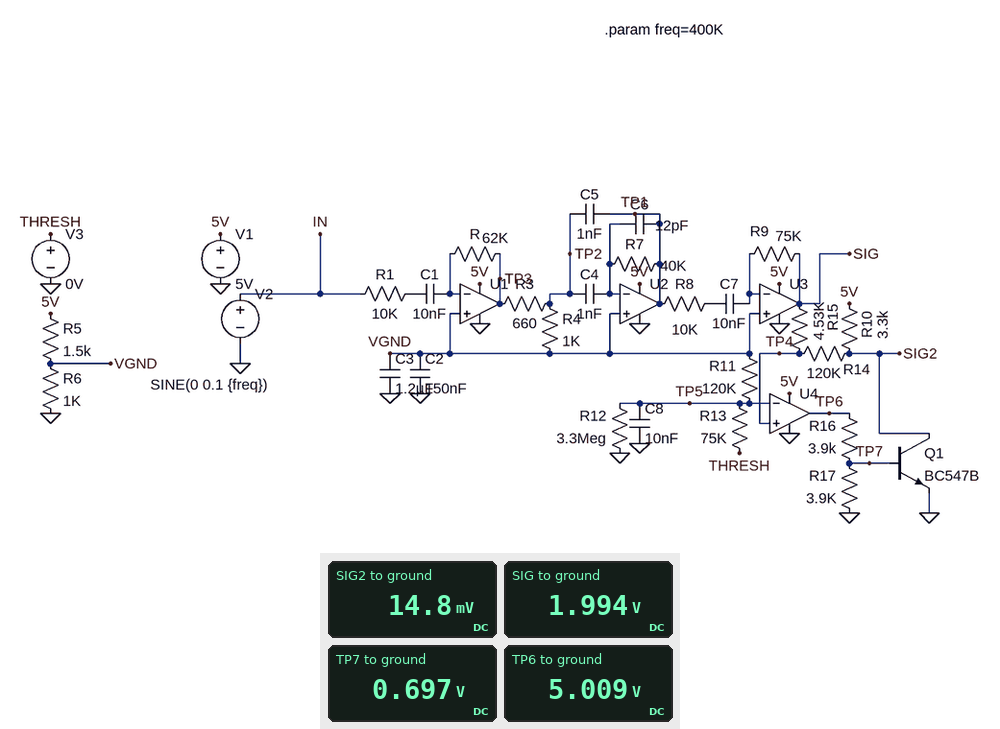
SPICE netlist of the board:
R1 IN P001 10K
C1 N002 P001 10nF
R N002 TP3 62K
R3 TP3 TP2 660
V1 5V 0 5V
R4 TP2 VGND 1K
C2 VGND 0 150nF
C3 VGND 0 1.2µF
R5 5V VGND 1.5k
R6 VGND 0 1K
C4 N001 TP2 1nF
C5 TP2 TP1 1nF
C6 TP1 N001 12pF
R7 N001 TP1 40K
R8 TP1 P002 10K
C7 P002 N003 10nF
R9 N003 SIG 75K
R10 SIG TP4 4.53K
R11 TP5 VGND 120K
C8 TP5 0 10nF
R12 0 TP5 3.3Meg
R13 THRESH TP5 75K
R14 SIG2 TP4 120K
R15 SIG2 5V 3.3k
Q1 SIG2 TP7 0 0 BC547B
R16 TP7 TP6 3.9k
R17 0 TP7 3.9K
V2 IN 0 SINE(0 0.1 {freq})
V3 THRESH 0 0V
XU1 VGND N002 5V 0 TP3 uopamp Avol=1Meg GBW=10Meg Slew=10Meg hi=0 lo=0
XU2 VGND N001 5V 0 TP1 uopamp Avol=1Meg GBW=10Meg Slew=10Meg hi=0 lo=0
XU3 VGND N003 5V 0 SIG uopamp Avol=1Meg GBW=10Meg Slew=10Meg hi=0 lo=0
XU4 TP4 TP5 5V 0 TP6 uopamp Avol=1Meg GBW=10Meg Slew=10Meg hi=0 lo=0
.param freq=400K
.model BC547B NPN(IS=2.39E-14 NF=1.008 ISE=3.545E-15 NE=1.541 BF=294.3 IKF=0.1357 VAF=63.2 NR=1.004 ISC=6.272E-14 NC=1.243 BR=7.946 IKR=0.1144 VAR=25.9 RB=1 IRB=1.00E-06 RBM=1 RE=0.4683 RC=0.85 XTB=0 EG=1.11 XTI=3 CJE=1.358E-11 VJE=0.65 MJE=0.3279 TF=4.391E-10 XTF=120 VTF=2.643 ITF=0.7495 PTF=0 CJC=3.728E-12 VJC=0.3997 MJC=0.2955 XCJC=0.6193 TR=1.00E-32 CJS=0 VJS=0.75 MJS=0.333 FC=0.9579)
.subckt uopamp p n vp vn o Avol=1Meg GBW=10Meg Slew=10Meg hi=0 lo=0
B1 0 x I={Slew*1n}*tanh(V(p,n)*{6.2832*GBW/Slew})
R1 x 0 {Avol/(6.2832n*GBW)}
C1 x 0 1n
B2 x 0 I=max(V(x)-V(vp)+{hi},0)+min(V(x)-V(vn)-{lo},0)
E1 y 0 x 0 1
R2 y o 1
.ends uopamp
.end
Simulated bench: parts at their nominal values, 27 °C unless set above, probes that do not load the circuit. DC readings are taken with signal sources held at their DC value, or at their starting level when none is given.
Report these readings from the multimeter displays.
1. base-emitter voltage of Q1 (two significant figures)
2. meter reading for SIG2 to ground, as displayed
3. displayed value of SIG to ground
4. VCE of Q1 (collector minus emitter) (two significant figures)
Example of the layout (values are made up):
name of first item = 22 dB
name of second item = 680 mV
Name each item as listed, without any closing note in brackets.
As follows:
base-emitter voltage of Q1 = 700 mV
meter reading for SIG2 to ground, as displayed = 14.8 mV
displayed value of SIG to ground = 1.994 V
VCE of Q1 (collector minus emitter) = 15 mV
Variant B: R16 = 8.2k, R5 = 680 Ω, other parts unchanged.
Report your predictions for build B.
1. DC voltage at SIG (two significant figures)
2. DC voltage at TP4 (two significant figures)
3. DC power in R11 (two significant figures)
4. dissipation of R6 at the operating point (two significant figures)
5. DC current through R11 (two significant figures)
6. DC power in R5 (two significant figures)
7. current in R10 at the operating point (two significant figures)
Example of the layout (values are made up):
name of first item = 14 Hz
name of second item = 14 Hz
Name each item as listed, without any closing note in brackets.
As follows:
DC voltage at SIG = 3.0 V
DC voltage at TP4 = 2.9 V
DC power in R11 = 28 µW
dissipation of R6 at the operating point = 8.8 mW
DC current through R11 = 15 µA
DC power in R5 = 6.1 mW
current in R10 at the operating point = 24 µA
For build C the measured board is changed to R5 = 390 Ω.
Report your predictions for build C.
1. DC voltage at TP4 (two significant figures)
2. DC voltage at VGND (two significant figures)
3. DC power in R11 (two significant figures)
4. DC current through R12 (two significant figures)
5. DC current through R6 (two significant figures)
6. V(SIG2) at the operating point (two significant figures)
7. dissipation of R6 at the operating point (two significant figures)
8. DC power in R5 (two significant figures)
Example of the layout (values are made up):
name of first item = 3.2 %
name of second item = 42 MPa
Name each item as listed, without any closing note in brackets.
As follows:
DC voltage at TP4 = 3.5 V
DC voltage at VGND = 3.6 V
DC power in R11 = 41 µW
DC current through R12 = 410 nA
DC current through R6 = 3.6 mA
V(SIG2) at the operating point = 15 mV
dissipation of R6 at the operating point = 13 mW
DC power in R5 = 5.1 mW
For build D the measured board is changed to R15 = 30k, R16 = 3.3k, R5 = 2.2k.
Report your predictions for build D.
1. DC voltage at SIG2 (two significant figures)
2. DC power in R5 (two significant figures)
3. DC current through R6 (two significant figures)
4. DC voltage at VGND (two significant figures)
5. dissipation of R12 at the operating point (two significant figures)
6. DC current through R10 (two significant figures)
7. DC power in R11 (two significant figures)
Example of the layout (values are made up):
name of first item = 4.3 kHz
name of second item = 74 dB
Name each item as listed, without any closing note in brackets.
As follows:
DC voltage at SIG2 = 8.1 mV
DC power in R5 = 5.4 mW
DC current through R6 = 1.6 mA
DC voltage at VGND = 1.6 V
dissipation of R12 at the operating point = 110 nW
DC current through R10 = 12 µA
DC power in R11 = 7.8 µW
